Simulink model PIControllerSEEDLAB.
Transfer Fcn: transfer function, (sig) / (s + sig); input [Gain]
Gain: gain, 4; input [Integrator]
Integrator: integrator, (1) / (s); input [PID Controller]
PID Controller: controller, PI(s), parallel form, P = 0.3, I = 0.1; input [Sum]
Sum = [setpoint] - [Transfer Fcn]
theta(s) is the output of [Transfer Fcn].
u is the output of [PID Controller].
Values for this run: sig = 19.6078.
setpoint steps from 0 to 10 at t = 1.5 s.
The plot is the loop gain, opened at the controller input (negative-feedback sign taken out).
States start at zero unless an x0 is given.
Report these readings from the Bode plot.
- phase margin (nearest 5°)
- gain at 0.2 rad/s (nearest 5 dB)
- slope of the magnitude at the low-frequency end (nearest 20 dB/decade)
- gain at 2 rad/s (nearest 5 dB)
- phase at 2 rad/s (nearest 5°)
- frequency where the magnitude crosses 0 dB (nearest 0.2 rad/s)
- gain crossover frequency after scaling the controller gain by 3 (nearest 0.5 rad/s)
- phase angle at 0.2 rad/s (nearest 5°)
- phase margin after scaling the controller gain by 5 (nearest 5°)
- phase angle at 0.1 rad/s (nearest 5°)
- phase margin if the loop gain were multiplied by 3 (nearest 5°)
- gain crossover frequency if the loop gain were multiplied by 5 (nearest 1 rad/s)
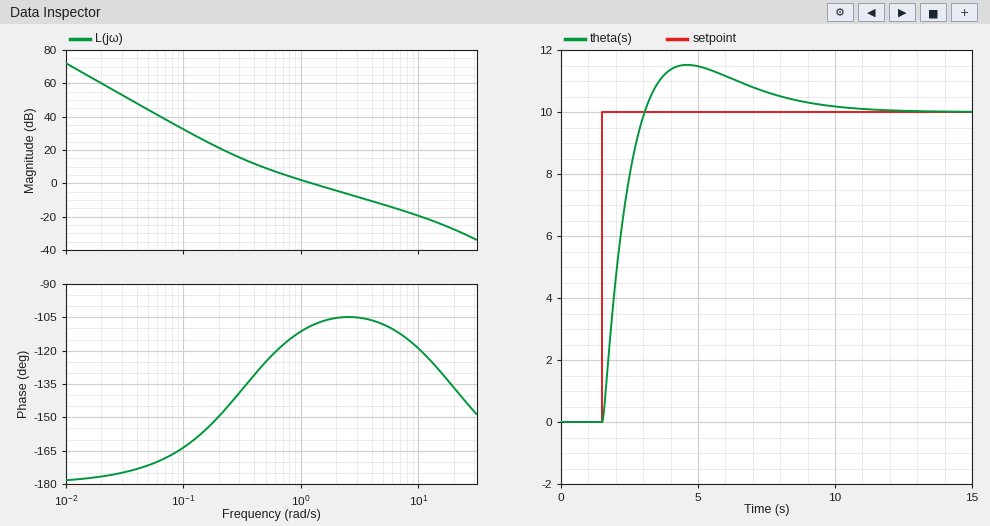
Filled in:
70°
20 dB
-40 dB/decade
-5 dB
-105°
1.2 rad/s
3.5 rad/s
-150°
70°
-165°
75°
6 rad/s
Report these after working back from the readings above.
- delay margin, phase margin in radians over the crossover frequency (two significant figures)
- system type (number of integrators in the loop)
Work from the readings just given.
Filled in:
1.0 s
2
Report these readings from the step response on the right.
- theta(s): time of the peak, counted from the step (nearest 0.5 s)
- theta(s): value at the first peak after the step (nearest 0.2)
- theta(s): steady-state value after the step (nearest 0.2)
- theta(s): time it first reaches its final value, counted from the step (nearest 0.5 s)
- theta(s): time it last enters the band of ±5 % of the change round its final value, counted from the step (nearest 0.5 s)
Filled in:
3.0 s
11.6
10.0
1.5 s
6.5 s
